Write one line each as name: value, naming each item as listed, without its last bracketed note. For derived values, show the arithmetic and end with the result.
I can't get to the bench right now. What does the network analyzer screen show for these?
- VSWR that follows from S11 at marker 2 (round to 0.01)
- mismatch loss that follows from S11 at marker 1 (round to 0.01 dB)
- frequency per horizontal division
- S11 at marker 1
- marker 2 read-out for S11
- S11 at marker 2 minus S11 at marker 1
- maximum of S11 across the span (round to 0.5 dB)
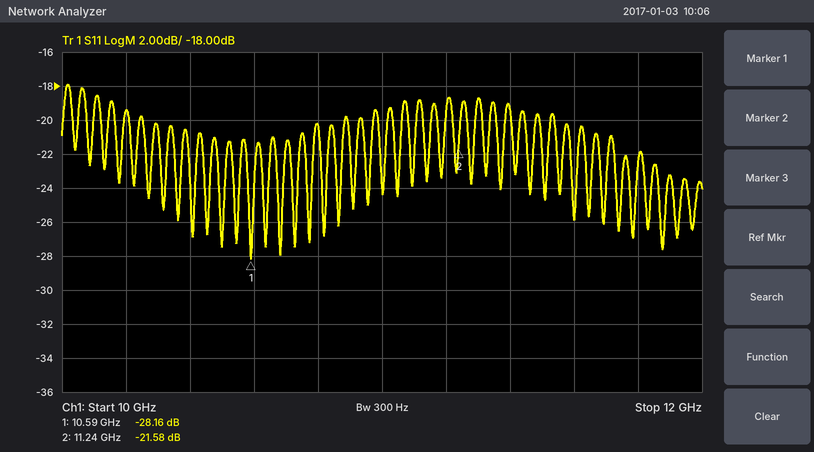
VSWR that follows from S11 at marker 2: (1 + 0.0834)/(1 − 0.0834) ≈ 1.18
mismatch loss that follows from S11 at marker 1: −10 log10(1 − 10^(-28.16/10)) ≈ 0.01 dB
frequency per horizontal division: 200 MHz
S11 at marker 1: -28.16 dB
marker 2 read-out for S11: -21.58 dB
S11 at marker 2 minus S11 at marker 1: -21.58 − (-28.16) = 6.58 dB
maximum of S11 across the span: -18.0 dB
